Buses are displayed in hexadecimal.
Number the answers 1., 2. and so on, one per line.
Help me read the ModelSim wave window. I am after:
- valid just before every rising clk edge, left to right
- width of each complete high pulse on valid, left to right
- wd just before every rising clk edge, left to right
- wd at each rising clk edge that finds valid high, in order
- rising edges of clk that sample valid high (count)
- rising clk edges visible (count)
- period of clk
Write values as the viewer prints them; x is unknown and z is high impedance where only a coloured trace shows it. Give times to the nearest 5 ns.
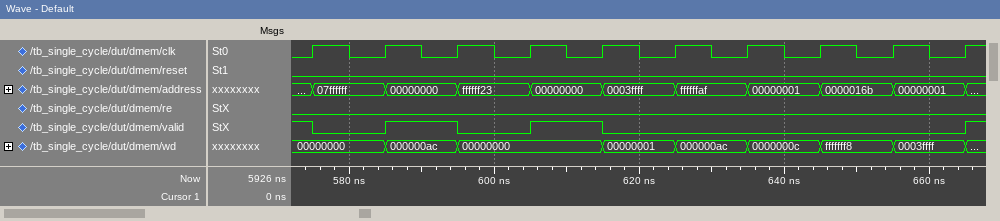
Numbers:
1. 1 0 1 0 1 0 0 0 0 0
2. 10 ns, 10 ns
3. 00000000, 00000000, 000000ac, 00000000, 00000000, 00000001, 000000ac, 0000000c, fffffff8, 0003ffff
4. 00000000, 000000ac, 00000000
5. 3
6. 10
7. 10 ns
